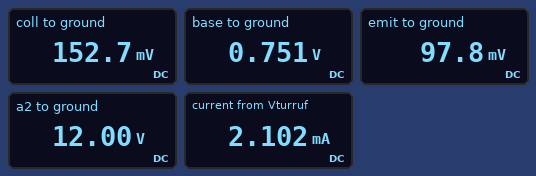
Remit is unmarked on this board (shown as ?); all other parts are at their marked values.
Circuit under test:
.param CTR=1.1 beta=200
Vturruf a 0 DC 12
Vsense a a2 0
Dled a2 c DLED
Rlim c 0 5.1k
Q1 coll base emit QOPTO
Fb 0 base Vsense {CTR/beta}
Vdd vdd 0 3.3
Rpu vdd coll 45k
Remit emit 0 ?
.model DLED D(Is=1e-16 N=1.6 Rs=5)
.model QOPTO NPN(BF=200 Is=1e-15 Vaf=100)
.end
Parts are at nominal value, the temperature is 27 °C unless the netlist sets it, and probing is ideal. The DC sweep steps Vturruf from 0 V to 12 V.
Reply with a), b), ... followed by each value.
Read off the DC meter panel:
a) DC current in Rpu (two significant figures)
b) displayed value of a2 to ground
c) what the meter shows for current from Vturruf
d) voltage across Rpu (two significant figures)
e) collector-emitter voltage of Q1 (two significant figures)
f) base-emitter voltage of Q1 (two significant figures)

a) 70 µA
b) 12.00 V
c) 2.102 mA
d) 3.1 V
e) 55 mV
f) 650 mV
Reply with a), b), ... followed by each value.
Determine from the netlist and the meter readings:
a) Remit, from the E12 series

a) 1.2 kΩ
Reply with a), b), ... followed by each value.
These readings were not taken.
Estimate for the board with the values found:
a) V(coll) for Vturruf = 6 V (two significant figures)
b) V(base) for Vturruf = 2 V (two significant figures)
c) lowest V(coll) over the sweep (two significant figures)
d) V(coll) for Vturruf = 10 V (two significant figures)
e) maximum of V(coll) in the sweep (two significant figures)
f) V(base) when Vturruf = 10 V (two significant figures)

a) 160 mV
b) 730 mV
c) 150 mV
d) 150 mV
e) 3.3 V
f) 750 mV
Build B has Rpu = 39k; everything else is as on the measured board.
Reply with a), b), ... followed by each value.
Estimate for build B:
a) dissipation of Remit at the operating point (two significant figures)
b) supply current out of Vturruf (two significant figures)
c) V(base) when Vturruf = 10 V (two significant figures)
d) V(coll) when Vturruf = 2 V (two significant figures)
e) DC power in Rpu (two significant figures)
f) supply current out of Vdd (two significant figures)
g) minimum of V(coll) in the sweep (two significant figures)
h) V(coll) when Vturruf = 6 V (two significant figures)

a) 10 µW
b) 2.1 mA
c) 760 mV
d) 230 mV
e) 250 µW
f) 80 µA
g) 170 mV
h) 180 mV
